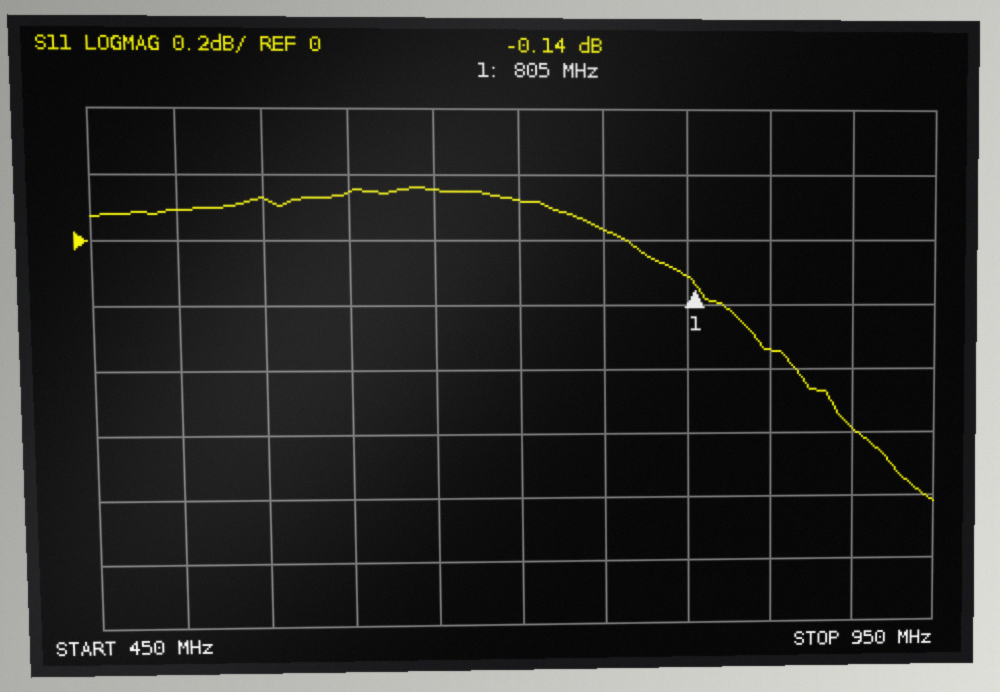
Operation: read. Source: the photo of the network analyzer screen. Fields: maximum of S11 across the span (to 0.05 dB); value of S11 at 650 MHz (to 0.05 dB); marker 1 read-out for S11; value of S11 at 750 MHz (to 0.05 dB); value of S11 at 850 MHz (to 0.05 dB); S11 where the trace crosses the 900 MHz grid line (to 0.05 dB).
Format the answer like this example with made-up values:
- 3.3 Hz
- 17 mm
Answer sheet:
- 0.15 dB
- 0.15 dB
- -0.14 dB
- 0.05 dB
- -0.35 dB
- -0.60 dB
